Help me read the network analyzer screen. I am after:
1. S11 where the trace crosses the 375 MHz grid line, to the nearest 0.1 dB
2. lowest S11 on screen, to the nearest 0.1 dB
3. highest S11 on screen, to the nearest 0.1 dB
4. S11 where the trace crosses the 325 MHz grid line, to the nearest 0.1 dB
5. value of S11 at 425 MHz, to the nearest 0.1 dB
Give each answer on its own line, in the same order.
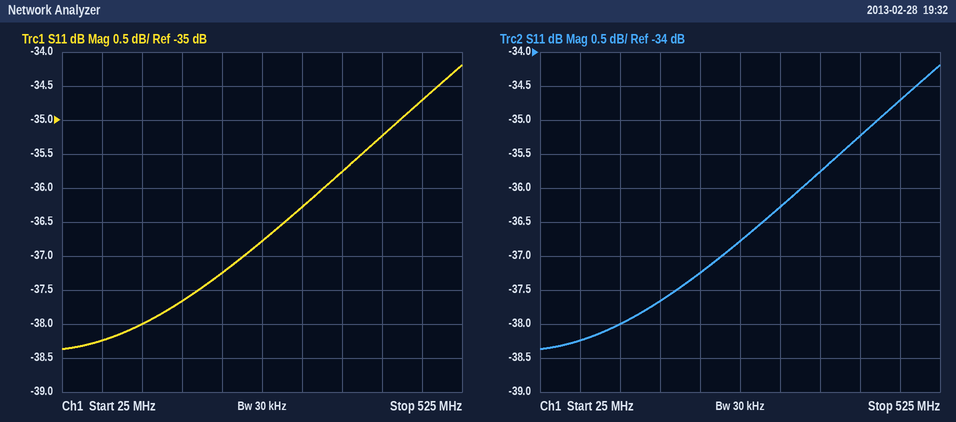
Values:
-35.8 dB
-38.4 dB
-34.2 dB
-36.3 dB
-35.2 dB
